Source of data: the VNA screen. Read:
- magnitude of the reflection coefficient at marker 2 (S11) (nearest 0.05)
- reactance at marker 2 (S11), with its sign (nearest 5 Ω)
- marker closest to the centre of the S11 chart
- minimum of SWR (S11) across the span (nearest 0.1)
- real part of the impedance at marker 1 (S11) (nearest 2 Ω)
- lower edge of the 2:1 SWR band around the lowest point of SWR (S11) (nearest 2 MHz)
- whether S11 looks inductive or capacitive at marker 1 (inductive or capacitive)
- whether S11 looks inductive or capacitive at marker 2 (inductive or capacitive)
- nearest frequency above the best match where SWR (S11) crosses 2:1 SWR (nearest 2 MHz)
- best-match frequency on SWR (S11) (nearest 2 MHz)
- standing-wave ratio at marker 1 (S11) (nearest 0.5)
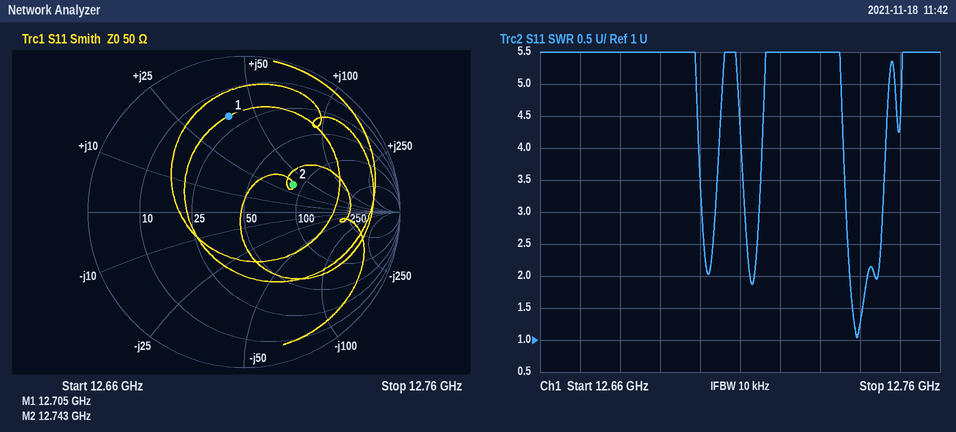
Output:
0.35
+35 Ω
marker 2
1.0
20 Ω
12.738 GHz
inductive
inductive
12.742 GHz
12.740 GHz
4.5
